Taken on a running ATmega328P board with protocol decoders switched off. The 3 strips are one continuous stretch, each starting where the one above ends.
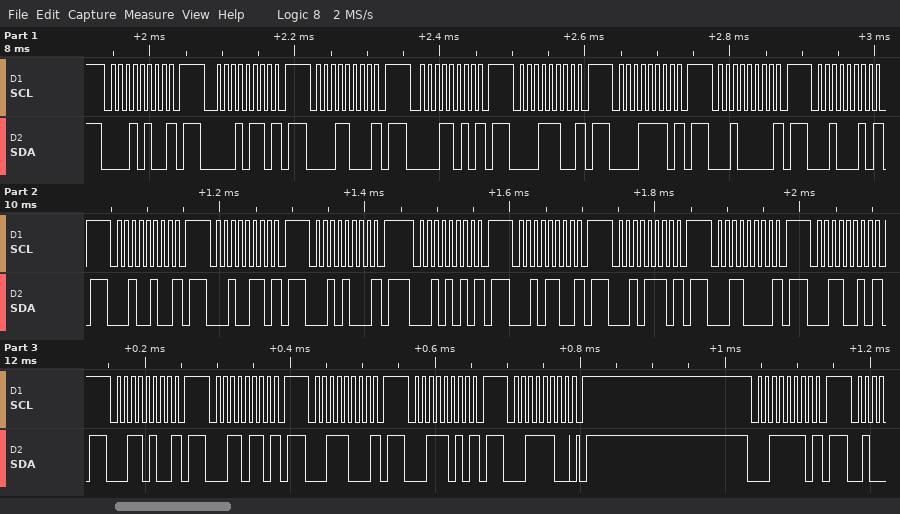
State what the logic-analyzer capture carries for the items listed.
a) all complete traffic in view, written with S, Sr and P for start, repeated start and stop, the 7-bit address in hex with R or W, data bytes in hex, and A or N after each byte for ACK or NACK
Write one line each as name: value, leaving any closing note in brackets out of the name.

all complete traffic in view, written with S, Sr and P for start, repeated start and stop, the 7-bit address in hex with R or W, data bytes in hex, and A or N after each byte for ACK or NACK: S 0AW N P S 0BW N P S 0CW N P S 0DW N P S 0EW N P S 0FW N P S 10W N P S 11W N P S 12W N P S 13W N P S 14W N P S 15W N P S 16W N P S 17W N P S 18W N P S 19W N P S 1AW N P S 1BW N P S 1CW N P S 1DW N P S 1EW A P S 1FW N P
